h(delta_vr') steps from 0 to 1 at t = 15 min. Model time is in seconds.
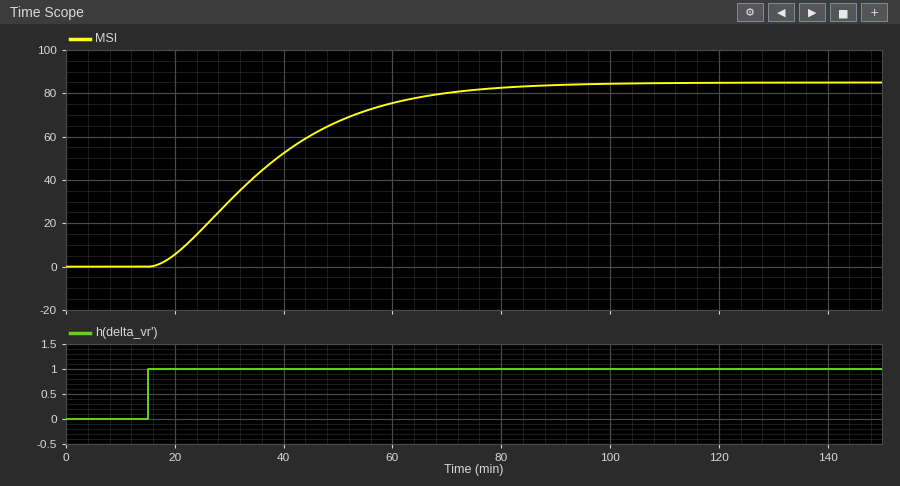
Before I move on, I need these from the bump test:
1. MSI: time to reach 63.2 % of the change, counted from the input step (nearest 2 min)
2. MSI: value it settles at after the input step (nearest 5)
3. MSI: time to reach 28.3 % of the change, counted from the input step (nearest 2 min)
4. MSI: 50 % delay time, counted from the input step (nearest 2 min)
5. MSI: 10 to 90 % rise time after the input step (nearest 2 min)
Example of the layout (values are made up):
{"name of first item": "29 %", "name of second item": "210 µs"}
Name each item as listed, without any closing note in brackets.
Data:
{"MSI: time to reach 63.2 % of the change, counted from the input step": "26 min", "MSI: value it settles at after the input step": "85", "MSI: time to reach 28.3 % of the change, counted from the input step": "12 min", "MSI: 50 % delay time, counted from the input step": "20 min", "MSI: 10 to 90 % rise time after the input step": "40 min"}
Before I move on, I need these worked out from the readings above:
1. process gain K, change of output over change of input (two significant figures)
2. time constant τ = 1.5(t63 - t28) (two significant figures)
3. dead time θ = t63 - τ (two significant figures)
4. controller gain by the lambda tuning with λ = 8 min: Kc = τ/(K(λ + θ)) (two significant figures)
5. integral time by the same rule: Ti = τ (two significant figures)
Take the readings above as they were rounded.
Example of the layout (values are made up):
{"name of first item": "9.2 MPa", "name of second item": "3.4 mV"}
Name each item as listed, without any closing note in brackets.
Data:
{"process gain K, change of output over change of input": "85", "time constant τ = 1.5(t63 - t28)": "21 min", "dead time θ = t63 - τ": "5.0 min", "controller gain by the lambda tuning with λ = 8 min: Kc = τ/(K(λ + θ))": "0.019", "integral time by the same rule: Ti = τ": "21 min"}
